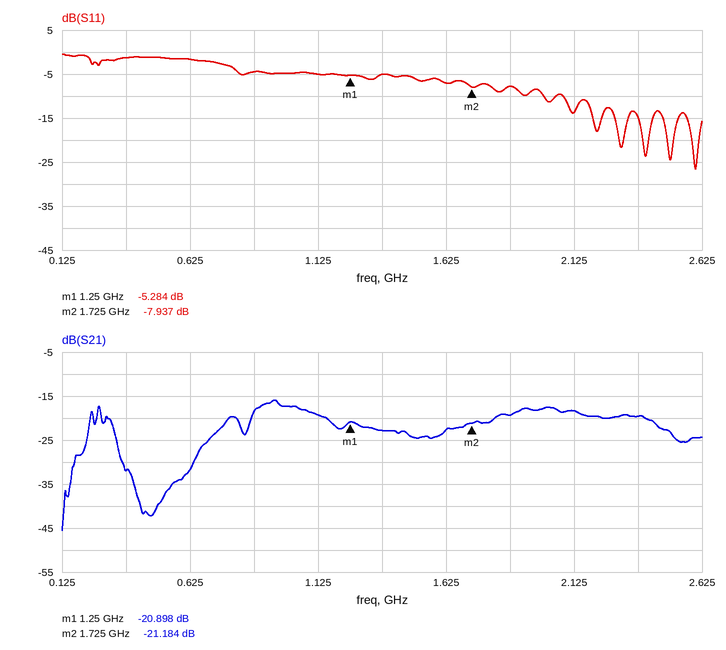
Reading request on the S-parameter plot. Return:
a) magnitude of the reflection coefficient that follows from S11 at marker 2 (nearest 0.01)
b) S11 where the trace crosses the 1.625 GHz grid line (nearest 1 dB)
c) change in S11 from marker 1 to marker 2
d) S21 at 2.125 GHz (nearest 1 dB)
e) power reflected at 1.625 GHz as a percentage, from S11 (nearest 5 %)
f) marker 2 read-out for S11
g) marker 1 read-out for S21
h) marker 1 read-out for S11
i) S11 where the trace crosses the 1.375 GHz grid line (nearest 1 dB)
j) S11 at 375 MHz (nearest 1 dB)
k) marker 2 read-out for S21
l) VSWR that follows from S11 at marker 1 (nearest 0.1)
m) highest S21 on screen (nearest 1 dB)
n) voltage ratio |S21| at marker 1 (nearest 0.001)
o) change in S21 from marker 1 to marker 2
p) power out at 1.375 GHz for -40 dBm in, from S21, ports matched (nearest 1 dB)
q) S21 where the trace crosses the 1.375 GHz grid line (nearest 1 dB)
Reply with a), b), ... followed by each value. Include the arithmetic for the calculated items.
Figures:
a) 10^(-7.937/20) ≈ 0.40
b) -7 dB
c) -7.937 − (-5.284) = -2.653 dB
d) -18 dB
e) 10^(-7/10) ≈ 20 %
f) -7.937 dB
g) -20.898 dB
h) -5.284 dB
i) -5 dB
j) -1 dB
k) -21.184 dB
l) (1 + 0.5443)/(1 − 0.5443) ≈ 3.4
m) -16 dB
n) 10^(-20.898/20) ≈ 0.090
o) -21.184 − (-20.898) = -0.286 dB
p) -40 dBm + (-23 dB) = -63 dBm
q) -23 dB
